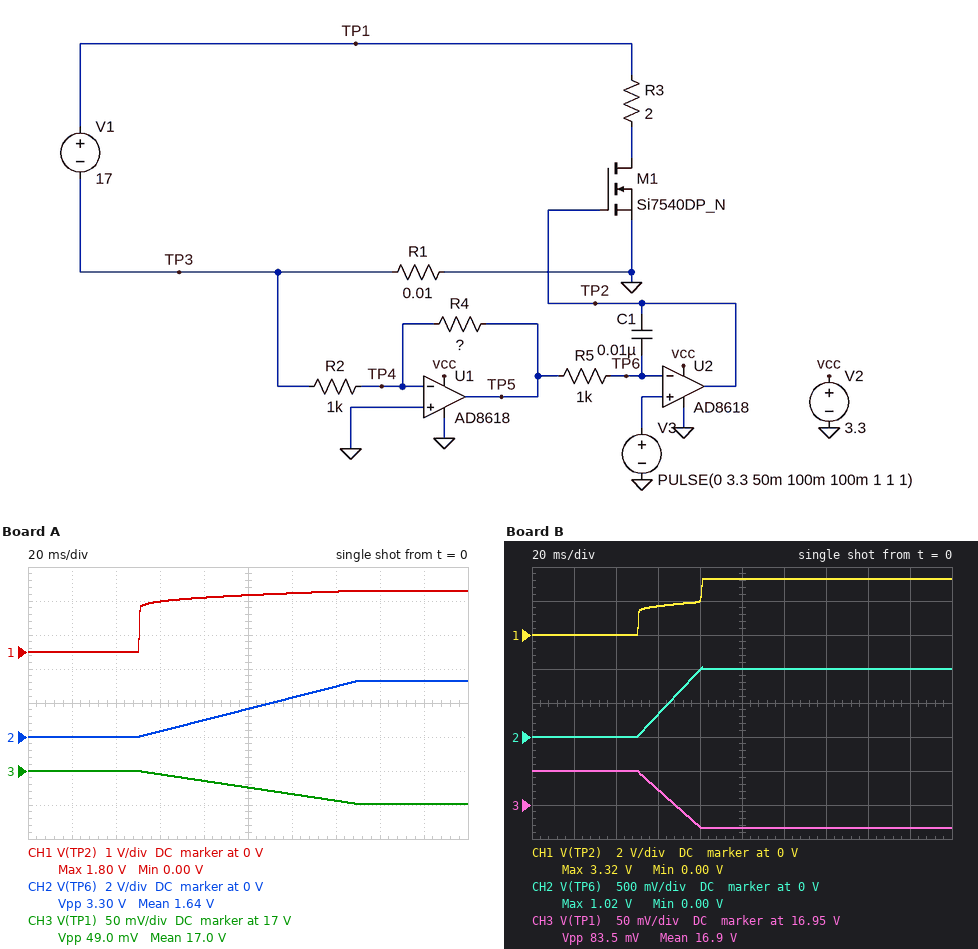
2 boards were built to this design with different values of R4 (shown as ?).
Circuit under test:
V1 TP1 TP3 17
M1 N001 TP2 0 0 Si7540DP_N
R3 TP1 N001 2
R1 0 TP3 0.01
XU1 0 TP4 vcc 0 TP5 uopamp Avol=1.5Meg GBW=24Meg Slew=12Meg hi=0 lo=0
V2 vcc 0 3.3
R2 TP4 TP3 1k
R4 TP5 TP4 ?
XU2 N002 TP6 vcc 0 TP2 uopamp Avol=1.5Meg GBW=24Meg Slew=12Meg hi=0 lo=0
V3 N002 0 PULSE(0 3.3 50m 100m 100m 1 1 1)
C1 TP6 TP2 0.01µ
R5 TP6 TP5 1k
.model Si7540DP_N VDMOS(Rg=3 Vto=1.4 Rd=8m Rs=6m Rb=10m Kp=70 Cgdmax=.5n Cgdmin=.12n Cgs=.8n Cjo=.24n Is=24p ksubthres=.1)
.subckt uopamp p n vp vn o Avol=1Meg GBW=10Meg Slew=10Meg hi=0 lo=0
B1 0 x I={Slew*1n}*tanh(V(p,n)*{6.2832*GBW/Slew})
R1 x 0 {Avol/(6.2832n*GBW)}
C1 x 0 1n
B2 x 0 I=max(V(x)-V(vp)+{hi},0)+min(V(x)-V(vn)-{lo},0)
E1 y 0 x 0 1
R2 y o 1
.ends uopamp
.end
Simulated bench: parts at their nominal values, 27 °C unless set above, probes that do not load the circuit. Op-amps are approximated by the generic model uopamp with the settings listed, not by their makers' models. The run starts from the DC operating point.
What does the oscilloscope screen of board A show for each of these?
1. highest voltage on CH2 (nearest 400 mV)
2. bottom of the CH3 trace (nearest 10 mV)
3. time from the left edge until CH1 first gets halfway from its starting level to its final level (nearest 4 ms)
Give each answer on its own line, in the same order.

3.2 V
16.95 V
52 ms
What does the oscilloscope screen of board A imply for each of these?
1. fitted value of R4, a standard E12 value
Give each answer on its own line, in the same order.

68 kΩ
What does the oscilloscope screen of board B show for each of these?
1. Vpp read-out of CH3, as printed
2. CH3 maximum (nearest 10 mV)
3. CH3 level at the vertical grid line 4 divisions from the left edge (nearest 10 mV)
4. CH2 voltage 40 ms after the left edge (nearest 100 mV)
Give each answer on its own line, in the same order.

83.5 mV
17.00 V
16.92 V
0 V
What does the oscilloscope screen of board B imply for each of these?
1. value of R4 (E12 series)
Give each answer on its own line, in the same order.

12 kΩ
